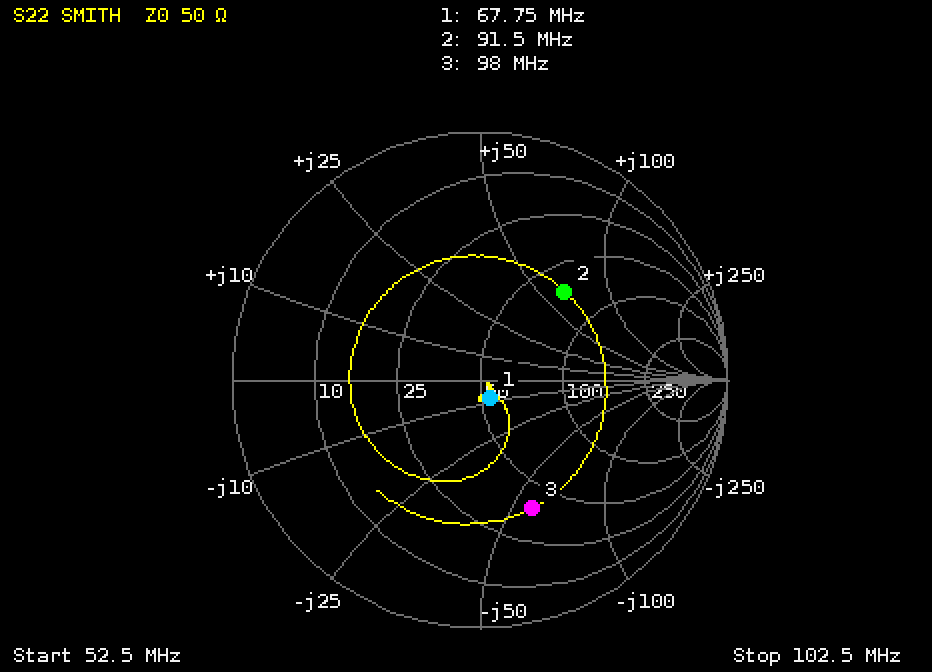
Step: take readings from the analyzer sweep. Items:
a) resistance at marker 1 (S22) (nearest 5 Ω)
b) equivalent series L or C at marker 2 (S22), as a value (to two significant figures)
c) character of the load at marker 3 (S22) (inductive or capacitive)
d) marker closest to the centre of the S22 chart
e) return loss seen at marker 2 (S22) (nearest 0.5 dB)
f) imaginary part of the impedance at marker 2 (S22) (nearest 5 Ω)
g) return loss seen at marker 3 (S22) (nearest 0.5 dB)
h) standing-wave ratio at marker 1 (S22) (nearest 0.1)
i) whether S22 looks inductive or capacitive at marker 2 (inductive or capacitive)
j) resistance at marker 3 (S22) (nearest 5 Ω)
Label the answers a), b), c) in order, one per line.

a) 55 Ω
b) 110 nH
c) capacitive
d) marker 1
e) 6.0 dB
f) +65 Ω
g) 5.0 dB
h) 1.2
i) inductive
j) 40 Ω
